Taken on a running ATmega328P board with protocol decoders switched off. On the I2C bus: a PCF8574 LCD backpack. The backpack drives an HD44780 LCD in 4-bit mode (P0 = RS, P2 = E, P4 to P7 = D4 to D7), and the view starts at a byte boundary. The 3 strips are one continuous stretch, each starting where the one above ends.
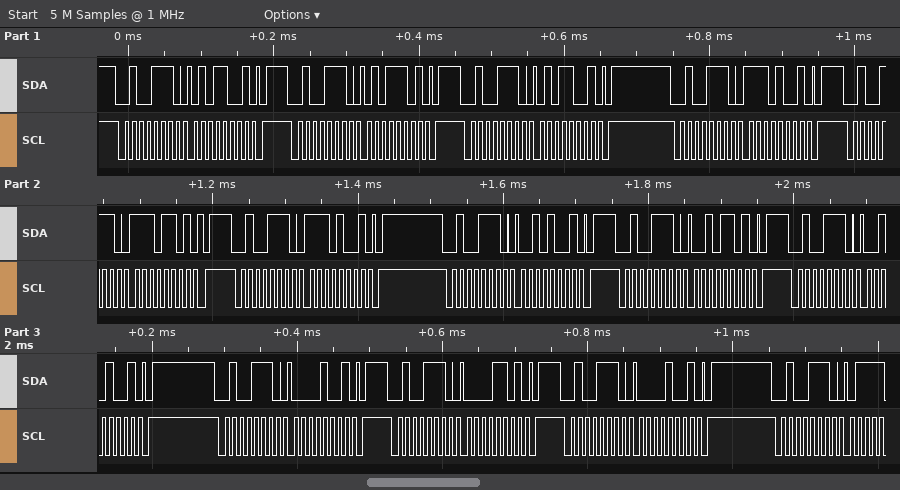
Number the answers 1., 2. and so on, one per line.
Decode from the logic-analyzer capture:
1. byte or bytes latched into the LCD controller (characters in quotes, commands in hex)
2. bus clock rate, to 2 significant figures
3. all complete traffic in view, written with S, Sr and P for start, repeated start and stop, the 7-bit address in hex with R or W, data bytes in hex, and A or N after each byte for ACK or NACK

1. '^' ' '
2. 100 kHz
3. S 27W A 59 A P S 27W A 5D A P S 27W A 59 A P S 27W A E9 A P S 27W A ED A P S 27W A E9 A P S 27W A 29 A P S 27W A 2D A P S 27W A 29 A P S 27W A 09 A P S 27W A 0D A P S 27W A 09 A P S 27W A
